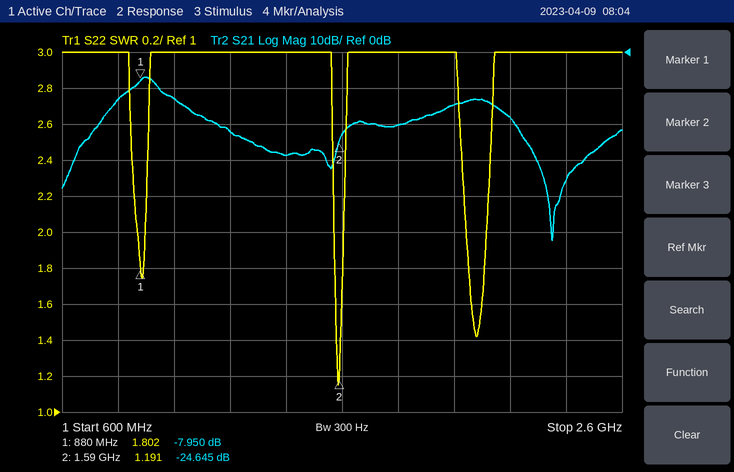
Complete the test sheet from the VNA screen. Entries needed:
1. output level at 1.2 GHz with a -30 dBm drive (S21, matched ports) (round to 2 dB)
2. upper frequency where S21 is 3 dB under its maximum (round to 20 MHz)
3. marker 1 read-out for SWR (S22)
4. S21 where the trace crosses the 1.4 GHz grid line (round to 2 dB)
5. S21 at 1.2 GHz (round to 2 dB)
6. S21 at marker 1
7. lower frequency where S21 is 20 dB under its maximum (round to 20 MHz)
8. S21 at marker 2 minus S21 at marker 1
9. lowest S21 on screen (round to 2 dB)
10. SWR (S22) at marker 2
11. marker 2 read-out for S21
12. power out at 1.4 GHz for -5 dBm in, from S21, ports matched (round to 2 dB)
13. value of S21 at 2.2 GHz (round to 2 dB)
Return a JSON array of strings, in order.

["-52 dBm", "940 MHz", "1.802", "-28 dB", "-22 dB", "-7.950 dB", "660 MHz", "-16.695 dB", "-52 dB", "1.191", "-24.645 dB", "-34 dBm", "-18 dB"]
